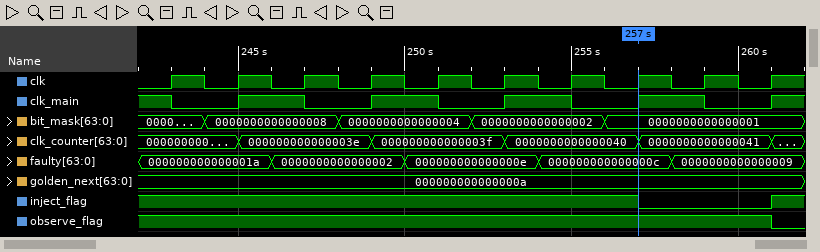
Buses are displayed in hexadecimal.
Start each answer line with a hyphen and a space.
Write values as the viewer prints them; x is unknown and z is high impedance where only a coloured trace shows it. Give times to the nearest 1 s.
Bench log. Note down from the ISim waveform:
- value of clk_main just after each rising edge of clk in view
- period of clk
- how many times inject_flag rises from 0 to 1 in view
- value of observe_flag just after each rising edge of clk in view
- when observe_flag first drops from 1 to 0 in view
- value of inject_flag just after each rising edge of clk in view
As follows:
- 0 1 0 1 0 1 0 1 0 1
- 2 s
- 1
- 1 1 1 1 1 1 1 1 1 0
- 261 s
- 1 1 1 1 1 1 1 0 0 1
